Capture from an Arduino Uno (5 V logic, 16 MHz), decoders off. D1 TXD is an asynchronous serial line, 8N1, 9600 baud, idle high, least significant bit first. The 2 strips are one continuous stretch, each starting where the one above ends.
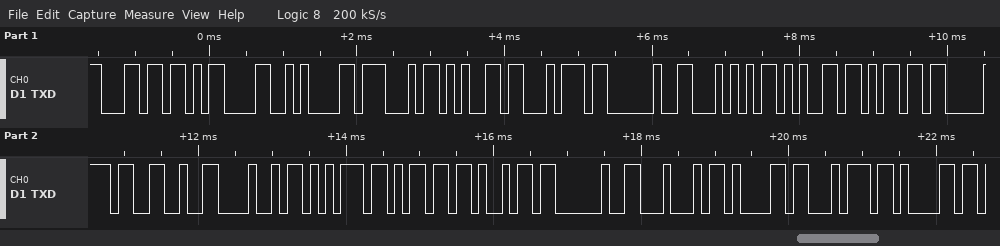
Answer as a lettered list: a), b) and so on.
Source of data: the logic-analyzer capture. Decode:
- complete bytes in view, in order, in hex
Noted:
a) 0x6C 0x0D 0x0A 0x47 0x65 0x74 0x20 0x54 0x65 0x6D 0x70 0x26 0x48 0x75 0x6D 0x69 0x20 0x44 0x61 0x74 0x61
